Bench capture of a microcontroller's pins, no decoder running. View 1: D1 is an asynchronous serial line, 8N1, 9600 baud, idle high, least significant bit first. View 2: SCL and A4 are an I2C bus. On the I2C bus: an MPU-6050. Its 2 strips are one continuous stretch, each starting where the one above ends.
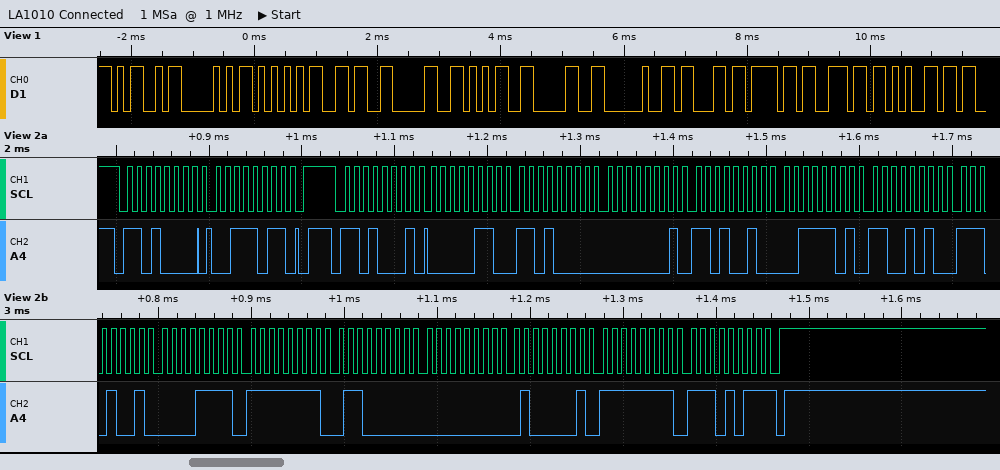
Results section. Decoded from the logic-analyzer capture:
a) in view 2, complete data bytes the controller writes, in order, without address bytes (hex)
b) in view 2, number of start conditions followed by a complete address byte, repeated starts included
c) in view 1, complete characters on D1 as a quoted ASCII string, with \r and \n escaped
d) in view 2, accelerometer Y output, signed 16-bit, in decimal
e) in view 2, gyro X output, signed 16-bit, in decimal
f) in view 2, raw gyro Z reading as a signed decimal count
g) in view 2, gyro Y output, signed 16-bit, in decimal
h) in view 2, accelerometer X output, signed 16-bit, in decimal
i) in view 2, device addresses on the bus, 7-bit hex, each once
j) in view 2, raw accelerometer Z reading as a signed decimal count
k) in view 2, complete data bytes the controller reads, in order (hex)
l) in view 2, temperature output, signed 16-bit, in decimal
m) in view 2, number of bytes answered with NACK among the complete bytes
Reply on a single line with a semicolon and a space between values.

3B; 2; "MPU6050 cone"; 466; -160; -21; 65; 1744; 0x68; 15818; 06 D0 01 D2 3D CA E9 0F FF 60 00 41 FF EB; -5873; 1
